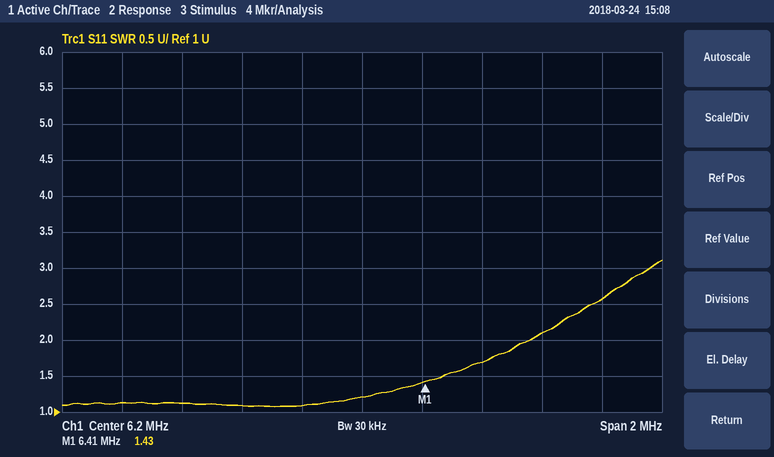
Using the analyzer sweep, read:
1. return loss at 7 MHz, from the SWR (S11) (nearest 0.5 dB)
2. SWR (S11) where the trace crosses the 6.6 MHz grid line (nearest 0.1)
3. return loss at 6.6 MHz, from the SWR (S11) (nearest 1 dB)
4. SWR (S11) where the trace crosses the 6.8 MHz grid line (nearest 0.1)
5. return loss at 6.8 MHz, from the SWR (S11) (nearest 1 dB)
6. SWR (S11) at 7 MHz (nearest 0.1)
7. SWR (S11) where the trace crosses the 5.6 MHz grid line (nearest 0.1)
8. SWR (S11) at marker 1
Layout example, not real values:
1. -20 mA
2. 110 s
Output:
1. 7.0 dB
2. 1.7
3. 12 dB
4. 2.1
5. 9 dB
6. 2.6
7. 1.1
8. 1.43
